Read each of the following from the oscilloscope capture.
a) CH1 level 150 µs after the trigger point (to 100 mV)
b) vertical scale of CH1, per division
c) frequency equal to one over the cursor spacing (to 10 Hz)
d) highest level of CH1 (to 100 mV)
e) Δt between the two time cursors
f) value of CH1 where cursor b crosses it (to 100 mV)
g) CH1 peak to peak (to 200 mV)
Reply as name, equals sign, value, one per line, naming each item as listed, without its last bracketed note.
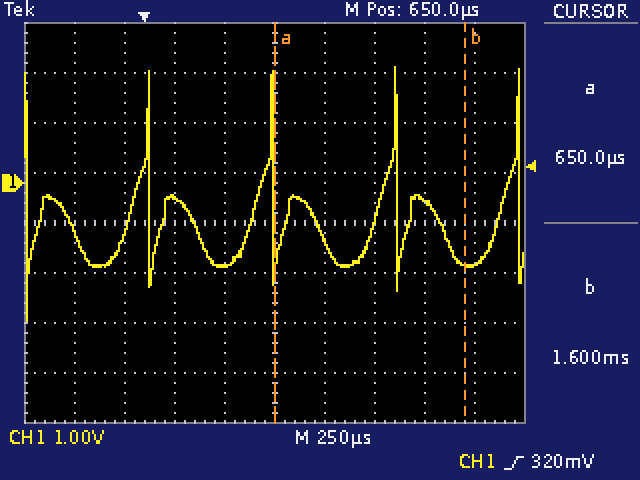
CH1 level 150 µs after the trigger point = -300 mV
vertical scale of CH1, per division = 1 V
frequency equal to one over the cursor spacing = 1.05 kHz
highest level of CH1 = 2.3 V
Δt between the two time cursors = 950 µs
value of CH1 where cursor b crosses it = -1.6 V
CH1 peak to peak = 5.0 V
